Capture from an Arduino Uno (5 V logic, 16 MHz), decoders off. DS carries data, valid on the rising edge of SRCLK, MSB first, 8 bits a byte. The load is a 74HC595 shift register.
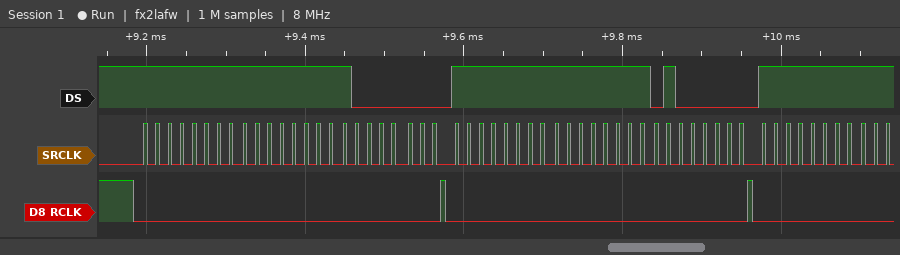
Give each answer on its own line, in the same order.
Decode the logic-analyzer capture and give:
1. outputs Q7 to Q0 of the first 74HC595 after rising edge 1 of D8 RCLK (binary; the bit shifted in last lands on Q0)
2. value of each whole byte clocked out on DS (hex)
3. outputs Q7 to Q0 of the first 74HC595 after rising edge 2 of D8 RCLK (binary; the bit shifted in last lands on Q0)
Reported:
10000000
FF FF 80 FF FF 40 FF
01000000
